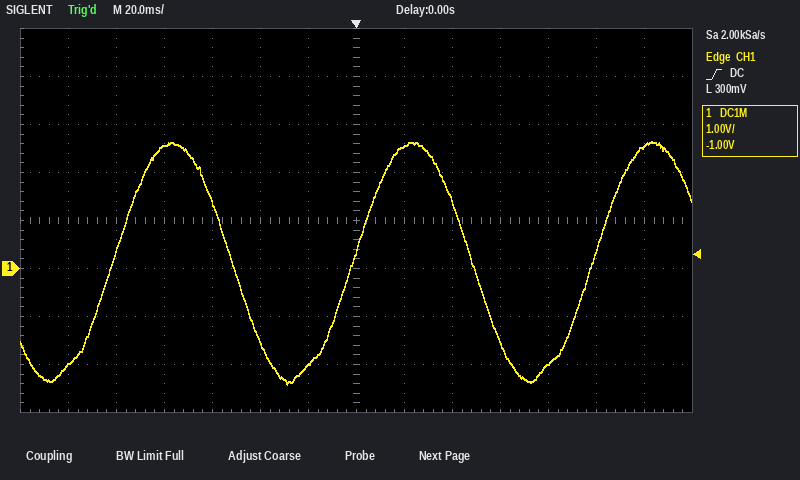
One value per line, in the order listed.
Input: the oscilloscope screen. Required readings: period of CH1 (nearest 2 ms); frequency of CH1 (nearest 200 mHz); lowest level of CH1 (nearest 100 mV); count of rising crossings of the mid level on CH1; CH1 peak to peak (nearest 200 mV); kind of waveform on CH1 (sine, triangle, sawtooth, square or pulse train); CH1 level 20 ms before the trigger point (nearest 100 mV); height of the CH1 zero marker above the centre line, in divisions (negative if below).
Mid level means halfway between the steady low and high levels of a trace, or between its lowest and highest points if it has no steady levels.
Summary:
100 ms
10.0 Hz
-2.4 V
3
5.0 V
sine
-2.0 V
-1.0 div
